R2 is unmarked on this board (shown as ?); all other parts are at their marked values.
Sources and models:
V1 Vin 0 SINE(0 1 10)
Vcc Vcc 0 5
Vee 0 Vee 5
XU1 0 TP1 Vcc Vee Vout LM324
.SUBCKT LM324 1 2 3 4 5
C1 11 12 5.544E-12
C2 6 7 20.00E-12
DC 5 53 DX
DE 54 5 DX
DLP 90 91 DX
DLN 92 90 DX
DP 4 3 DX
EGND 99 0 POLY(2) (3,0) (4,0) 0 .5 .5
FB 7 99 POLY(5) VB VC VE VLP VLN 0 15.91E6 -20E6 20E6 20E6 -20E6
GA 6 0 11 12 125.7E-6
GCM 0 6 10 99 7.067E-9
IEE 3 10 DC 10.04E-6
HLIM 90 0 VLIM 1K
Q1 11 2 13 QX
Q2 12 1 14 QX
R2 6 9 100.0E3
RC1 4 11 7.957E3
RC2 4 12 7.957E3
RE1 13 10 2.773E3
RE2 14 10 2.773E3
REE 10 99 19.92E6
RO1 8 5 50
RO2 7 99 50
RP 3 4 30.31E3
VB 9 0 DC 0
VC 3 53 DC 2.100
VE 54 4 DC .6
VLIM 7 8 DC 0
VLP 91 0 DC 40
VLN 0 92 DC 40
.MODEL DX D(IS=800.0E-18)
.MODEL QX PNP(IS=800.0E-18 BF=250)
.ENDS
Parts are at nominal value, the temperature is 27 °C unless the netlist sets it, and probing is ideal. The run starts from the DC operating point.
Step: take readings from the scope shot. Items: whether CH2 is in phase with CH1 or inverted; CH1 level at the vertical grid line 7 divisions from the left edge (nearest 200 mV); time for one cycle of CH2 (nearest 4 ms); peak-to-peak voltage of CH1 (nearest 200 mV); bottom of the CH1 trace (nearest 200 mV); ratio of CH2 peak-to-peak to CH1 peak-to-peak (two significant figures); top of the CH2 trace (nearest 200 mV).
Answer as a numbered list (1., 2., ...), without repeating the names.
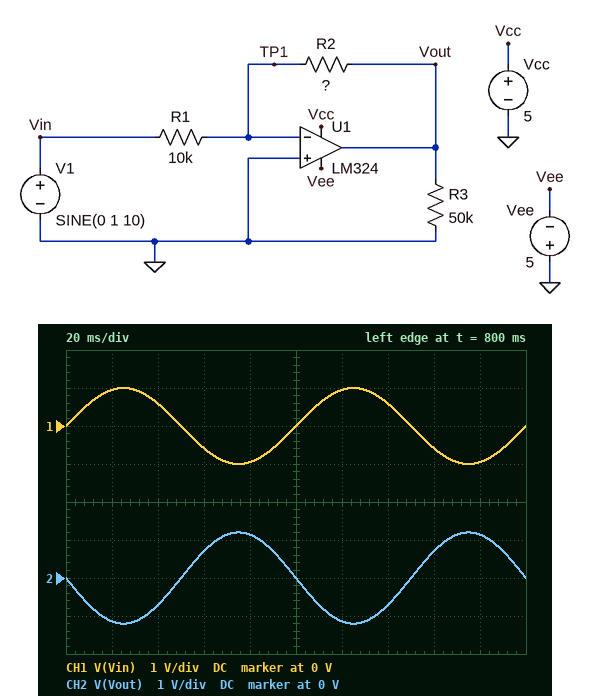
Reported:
1. inverted
2. 600 mV
3. 100 ms
4. 2.0 V
5. -1.0 V
6. 1.2
7. 1.2 V
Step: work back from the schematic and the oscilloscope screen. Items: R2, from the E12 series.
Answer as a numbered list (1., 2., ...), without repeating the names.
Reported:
1. 12 kΩ
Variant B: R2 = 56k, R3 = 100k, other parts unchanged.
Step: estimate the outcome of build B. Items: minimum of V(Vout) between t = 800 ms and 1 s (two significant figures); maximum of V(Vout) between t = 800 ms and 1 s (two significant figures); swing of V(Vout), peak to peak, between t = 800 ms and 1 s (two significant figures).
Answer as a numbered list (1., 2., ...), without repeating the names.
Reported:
1. -5.0 V
2. 3.5 V
3. 8.5 V
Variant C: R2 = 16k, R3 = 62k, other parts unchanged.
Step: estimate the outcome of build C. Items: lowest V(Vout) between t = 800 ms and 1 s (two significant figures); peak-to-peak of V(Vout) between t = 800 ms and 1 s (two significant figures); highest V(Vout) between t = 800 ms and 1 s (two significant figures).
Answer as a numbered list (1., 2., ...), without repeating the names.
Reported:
1. -1.6 V
2. 3.2 V
3. 1.6 V
